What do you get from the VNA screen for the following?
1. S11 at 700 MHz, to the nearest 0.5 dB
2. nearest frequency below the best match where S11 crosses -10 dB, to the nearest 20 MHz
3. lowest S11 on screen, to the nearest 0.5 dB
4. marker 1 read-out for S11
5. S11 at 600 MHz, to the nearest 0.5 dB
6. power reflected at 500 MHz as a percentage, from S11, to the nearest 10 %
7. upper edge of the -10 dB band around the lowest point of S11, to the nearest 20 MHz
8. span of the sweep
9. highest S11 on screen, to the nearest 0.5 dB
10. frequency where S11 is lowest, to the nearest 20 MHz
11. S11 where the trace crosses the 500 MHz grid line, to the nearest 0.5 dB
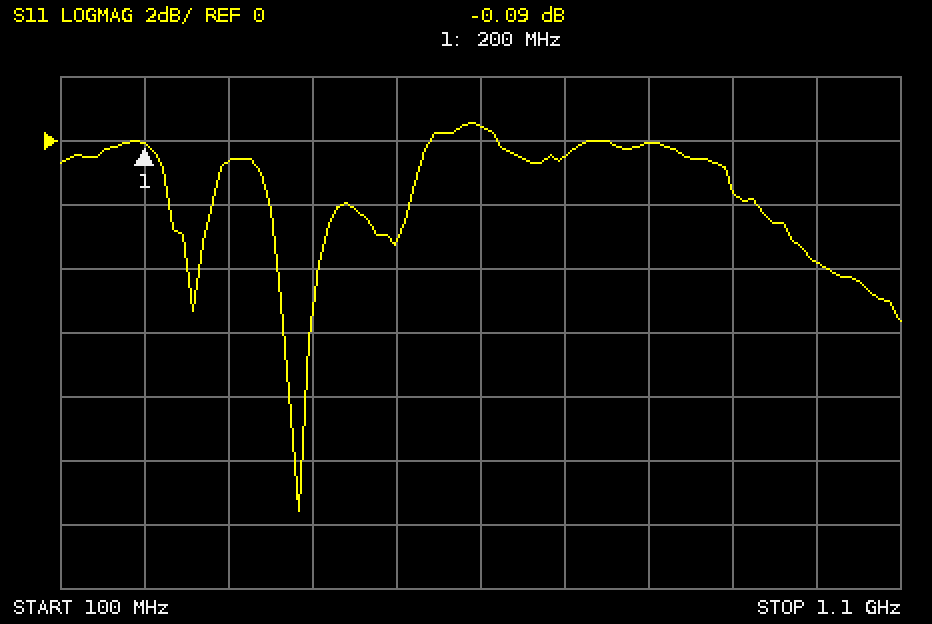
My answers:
-0.5 dB
380 MHz
-11.5 dB
-0.09 dB
0.5 dB
50 %
380 MHz
1 GHz
0.5 dB
380 MHz
-3.0 dB
